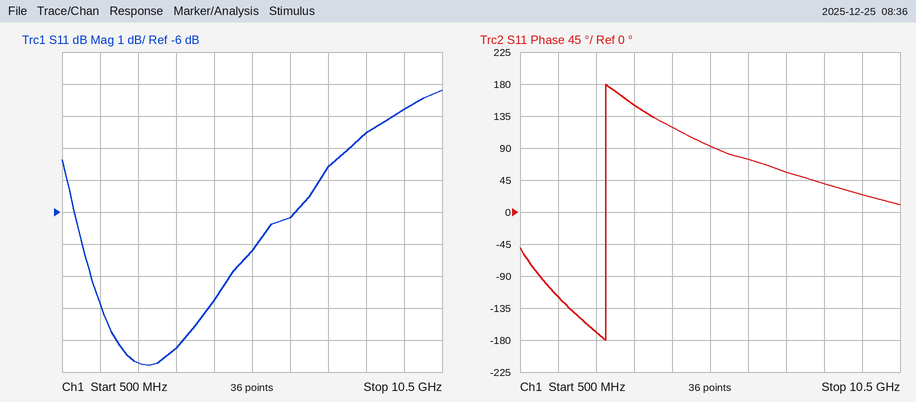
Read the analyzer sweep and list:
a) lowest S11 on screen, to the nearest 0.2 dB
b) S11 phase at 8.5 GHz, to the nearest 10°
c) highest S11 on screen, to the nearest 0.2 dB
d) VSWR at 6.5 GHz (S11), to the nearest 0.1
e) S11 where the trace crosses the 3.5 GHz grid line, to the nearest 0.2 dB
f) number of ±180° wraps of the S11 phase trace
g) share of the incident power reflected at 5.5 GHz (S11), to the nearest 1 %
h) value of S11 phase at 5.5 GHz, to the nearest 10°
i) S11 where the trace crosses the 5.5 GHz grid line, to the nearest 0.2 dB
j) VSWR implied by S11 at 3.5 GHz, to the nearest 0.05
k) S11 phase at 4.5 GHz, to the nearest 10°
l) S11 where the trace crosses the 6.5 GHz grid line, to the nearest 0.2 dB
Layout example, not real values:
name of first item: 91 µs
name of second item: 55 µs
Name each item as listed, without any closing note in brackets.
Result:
lowest S11 on screen, to the nearest 0.2 dB: -10.8 dB
S11 phase at 8.5 GHz, to the nearest 10°: 40°
highest S11 on screen, to the nearest 0.2 dB: -2.2 dB
VSWR at 6.5 GHz (S11), to the nearest 0.1: 2.9
S11 where the trace crosses the 3.5 GHz grid line, to the nearest 0.2 dB: -10.2 dB
number of ±180° wraps of the S11 phase trace: 1
share of the incident power reflected at 5.5 GHz (S11), to the nearest 1 %: 19 %
value of S11 phase at 5.5 GHz, to the nearest 10°: 90°
S11 where the trace crosses the 5.5 GHz grid line, to the nearest 0.2 dB: -7.2 dB
VSWR implied by S11 at 3.5 GHz, to the nearest 0.05: 1.90
S11 phase at 4.5 GHz, to the nearest 10°: 120°
S11 where the trace crosses the 6.5 GHz grid line, to the nearest 0.2 dB: -6.2 dB
